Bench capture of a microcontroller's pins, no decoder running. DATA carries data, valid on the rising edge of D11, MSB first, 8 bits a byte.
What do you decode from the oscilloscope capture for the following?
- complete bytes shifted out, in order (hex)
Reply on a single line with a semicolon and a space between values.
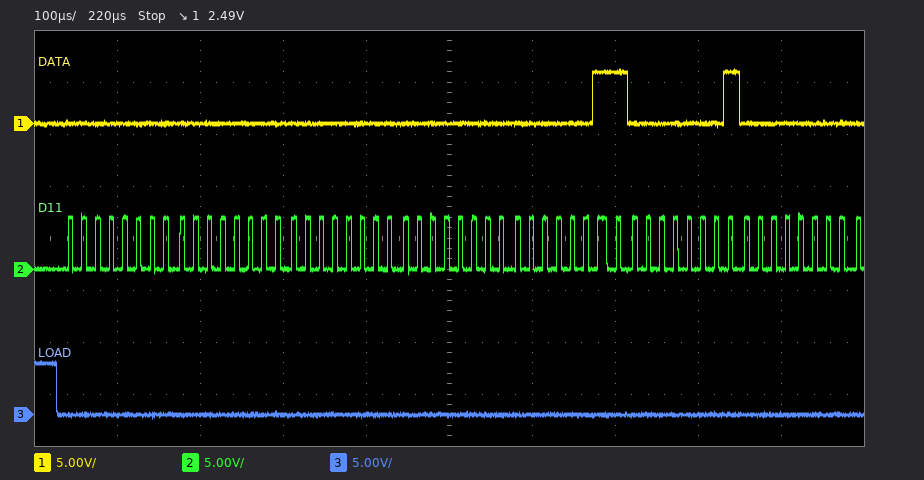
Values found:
00 00 00 00 03 01 00
